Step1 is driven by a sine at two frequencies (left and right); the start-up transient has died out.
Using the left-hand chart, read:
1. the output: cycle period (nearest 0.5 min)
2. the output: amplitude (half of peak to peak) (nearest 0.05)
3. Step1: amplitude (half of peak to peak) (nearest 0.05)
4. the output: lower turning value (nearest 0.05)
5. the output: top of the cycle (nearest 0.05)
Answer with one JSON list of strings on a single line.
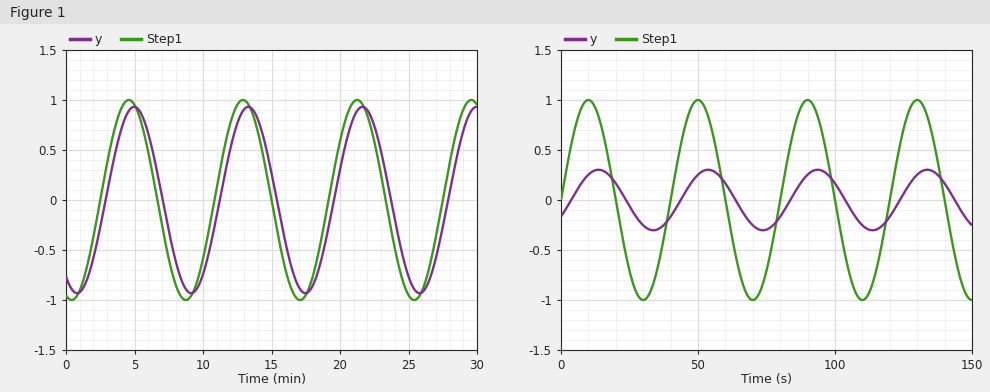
["8.5 min", "0.95", "1.00", "-0.95", "0.95"]
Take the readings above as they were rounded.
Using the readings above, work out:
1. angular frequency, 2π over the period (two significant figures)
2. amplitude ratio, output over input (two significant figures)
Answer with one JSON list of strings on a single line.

["0.74 rad/min", "0.95"]
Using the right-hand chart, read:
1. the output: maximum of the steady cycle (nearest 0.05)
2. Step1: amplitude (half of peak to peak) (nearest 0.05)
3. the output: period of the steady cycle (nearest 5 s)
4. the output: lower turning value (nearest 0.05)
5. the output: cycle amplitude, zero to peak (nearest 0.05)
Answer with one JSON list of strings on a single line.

["0.30", "1.00", "40 s", "-0.30", "0.30"]
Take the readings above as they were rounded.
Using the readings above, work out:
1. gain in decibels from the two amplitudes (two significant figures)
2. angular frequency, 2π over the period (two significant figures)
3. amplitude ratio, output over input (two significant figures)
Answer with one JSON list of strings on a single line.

["-10 dB", "0.16 rad/s", "0.30"]
